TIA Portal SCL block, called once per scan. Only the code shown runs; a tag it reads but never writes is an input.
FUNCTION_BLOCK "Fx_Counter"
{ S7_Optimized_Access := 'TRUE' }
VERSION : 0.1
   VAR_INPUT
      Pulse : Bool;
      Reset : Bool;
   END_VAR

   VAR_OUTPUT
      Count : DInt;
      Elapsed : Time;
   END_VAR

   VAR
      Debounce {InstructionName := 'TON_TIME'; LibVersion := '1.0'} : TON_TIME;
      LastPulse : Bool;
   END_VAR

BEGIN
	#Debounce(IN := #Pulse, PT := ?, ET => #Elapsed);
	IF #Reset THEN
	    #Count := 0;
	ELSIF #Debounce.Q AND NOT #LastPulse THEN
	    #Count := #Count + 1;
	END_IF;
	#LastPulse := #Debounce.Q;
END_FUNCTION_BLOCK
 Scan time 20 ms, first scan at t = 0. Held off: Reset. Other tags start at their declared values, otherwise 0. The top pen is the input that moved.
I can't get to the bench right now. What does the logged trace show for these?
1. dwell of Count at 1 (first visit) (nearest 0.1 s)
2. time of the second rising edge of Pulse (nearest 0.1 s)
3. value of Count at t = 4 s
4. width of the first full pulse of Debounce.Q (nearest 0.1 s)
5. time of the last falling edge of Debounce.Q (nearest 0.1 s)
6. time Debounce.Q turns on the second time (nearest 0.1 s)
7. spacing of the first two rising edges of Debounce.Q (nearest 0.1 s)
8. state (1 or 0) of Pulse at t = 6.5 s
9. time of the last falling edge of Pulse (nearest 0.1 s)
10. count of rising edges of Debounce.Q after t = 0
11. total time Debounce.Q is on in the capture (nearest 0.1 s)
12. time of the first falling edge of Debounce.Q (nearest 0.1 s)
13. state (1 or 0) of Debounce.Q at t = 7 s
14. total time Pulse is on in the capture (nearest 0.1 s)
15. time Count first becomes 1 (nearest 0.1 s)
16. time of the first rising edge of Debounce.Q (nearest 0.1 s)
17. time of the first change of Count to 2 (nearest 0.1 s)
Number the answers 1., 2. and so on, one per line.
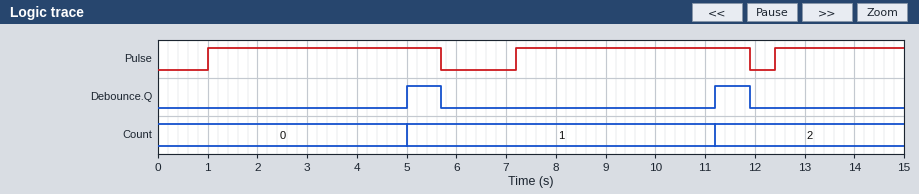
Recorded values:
1. 6.2 s
2. 7.2 s
3. 0
4. 0.7 s
5. 11.9 s
6. 11.2 s
7. 6.2 s
8. 0
9. 11.9 s
10. 2
11. 1.4 s
12. 5.7 s
13. 0
14. 12.0 s
15. 5.0 s
16. 5.0 s
17. 11.2 s
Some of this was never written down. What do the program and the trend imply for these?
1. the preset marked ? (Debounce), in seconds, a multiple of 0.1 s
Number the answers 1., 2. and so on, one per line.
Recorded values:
1. 4.0 s
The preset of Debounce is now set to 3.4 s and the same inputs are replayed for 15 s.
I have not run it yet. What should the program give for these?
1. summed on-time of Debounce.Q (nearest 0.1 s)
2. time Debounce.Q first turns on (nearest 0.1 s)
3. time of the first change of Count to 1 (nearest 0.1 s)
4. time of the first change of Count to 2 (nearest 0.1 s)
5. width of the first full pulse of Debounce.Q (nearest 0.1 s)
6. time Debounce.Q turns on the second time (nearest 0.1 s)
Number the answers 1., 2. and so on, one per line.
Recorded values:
1. 2.6 s
2. 4.4 s
3. 4.4 s
4. 10.6 s
5. 1.3 s
6. 10.6 s
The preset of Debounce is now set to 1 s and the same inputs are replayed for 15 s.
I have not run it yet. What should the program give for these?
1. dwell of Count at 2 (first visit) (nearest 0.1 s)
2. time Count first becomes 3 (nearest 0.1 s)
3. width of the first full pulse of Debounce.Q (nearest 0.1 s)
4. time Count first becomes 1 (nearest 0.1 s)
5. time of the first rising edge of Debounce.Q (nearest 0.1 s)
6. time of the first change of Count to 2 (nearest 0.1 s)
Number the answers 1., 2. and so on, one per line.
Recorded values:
1. 5.2 s
2. 13.4 s
3. 3.7 s
4. 2.0 s
5. 2.0 s
6. 8.2 s
